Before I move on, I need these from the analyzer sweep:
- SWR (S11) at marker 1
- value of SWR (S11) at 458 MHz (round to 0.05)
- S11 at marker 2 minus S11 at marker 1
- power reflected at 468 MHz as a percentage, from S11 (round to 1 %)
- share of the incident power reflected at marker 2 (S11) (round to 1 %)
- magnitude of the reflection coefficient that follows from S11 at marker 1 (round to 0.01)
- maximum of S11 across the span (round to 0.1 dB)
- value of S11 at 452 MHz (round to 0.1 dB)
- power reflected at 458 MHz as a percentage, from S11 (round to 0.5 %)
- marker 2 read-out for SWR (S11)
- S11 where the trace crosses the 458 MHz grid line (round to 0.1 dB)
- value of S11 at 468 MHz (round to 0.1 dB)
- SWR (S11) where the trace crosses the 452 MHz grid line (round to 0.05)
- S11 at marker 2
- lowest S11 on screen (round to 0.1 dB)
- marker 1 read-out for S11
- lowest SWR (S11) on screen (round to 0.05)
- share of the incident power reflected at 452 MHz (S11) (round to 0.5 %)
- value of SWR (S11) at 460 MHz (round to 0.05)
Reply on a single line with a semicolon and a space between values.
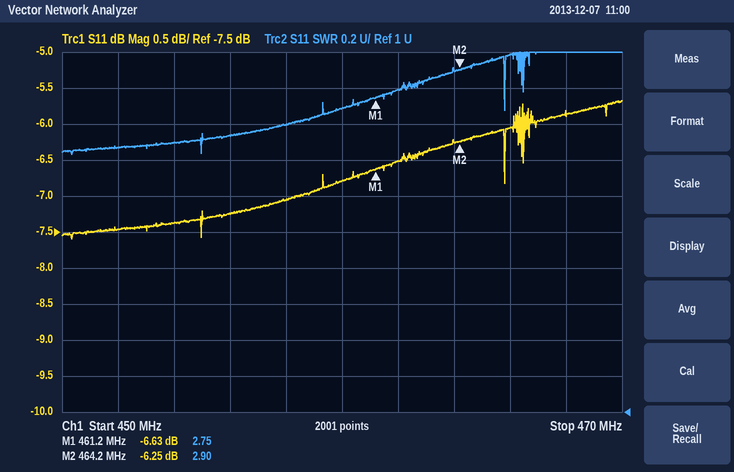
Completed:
2.75; 2.60; 0.38 dB; 26 %; 24 %; 0.47; -5.7 dB; -7.5 dB; 19.5 %; 2.90; -7.1 dB; -5.9 dB; 2.45; -6.25 dB; -7.6 dB; -6.63 dB; 2.45; 18.0 %; 2.70
